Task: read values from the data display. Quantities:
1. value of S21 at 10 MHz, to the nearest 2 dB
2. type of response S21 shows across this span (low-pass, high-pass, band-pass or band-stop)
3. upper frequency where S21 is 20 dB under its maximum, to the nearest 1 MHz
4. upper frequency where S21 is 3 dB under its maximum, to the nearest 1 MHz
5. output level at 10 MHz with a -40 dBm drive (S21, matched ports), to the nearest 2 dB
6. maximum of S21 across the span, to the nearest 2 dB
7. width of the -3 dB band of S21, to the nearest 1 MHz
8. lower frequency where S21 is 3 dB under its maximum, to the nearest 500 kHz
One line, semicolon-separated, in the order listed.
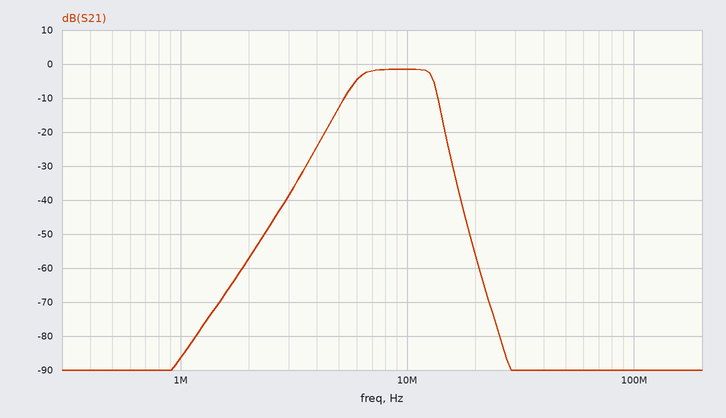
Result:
-2 dB; band-pass; 15 MHz; 13 MHz; -42 dBm; -2 dB; 7 MHz; 6.0 MHz
